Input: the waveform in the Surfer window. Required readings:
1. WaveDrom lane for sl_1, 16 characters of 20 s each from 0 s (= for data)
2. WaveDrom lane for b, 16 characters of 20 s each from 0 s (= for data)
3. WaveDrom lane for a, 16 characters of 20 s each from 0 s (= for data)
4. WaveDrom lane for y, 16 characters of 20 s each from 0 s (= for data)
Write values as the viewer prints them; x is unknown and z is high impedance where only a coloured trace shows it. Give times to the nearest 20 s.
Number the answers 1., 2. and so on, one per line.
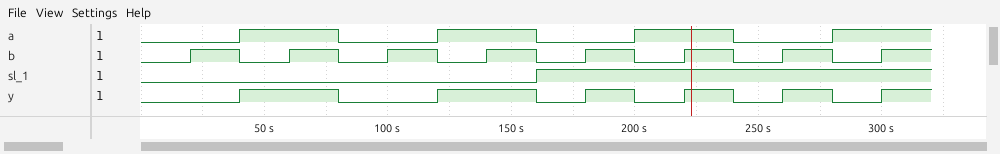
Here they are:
1. {name: 'sl_1', wave: '0.......1.......'}
2. {name: 'b', wave: '0101010101010101'}
3. {name: 'a', wave: '0.1.0.1.0.1.0.1.'}
4. {name: 'y', wave: '0.1.0.1.01010101'}
